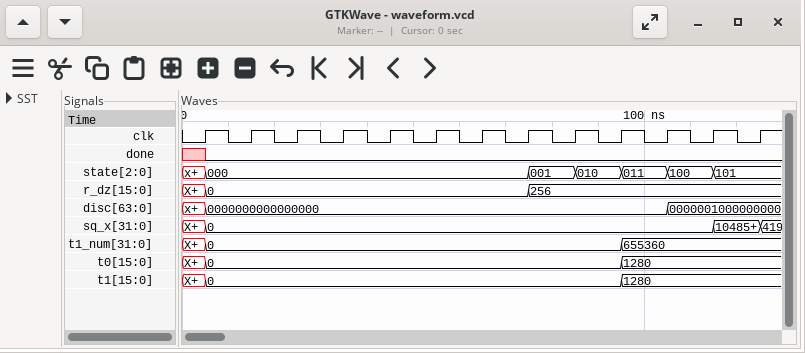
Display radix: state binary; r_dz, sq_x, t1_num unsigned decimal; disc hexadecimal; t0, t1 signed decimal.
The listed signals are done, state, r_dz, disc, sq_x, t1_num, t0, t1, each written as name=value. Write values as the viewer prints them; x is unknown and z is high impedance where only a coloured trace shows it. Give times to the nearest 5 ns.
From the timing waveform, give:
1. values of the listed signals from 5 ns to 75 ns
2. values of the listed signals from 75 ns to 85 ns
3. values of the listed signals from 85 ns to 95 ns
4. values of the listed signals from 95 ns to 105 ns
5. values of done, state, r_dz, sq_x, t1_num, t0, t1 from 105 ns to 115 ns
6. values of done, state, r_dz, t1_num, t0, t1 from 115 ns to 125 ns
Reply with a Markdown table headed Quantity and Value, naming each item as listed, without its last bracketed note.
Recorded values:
| Quantity | Value |
|---|---|
| values of the listed signals from 5 ns to 75 ns | done=0, state=000, r_dz=0, disc=0000000000000000, sq_x=0, t1_num=0, t0=0, t1=0 |
| values of the listed signals from 75 ns to 85 ns | done=0, state=001, r_dz=256, disc=0000000000000000, sq_x=0, t1_num=0, t0=0, t1=0 |
| values of the listed signals from 85 ns to 95 ns | done=0, state=010, r_dz=256, disc=0000000000000000, sq_x=0, t1_num=0, t0=0, t1=0 |
| values of the listed signals from 95 ns to 105 ns | done=0, state=011, r_dz=256, disc=0000000000000000, sq_x=0, t1_num=655360, t0=1280, t1=1280 |
| values of done, state, r_dz, sq_x, t1_num, t0, t1 from 105 ns to 115 ns | done=0, state=100, r_dz=256, sq_x=0, t1_num=655360, t0=1280, t1=1280 |
| values of done, state, r_dz, t1_num, t0, t1 from 115 ns to 125 ns | done=0, state=101, r_dz=256, t1_num=655360, t0=1280, t1=1280 |
